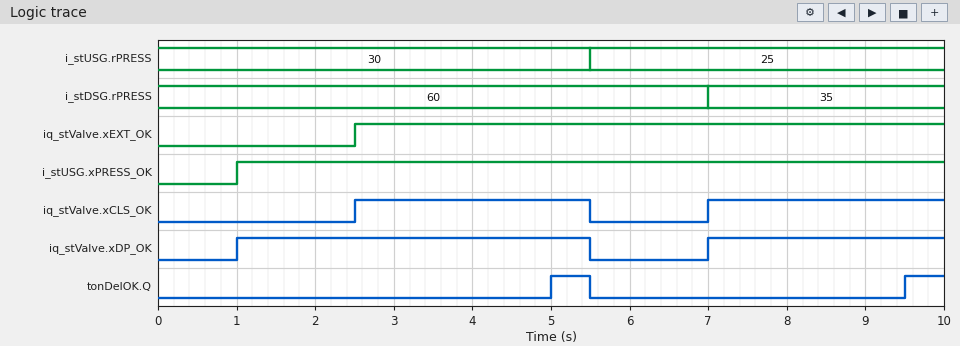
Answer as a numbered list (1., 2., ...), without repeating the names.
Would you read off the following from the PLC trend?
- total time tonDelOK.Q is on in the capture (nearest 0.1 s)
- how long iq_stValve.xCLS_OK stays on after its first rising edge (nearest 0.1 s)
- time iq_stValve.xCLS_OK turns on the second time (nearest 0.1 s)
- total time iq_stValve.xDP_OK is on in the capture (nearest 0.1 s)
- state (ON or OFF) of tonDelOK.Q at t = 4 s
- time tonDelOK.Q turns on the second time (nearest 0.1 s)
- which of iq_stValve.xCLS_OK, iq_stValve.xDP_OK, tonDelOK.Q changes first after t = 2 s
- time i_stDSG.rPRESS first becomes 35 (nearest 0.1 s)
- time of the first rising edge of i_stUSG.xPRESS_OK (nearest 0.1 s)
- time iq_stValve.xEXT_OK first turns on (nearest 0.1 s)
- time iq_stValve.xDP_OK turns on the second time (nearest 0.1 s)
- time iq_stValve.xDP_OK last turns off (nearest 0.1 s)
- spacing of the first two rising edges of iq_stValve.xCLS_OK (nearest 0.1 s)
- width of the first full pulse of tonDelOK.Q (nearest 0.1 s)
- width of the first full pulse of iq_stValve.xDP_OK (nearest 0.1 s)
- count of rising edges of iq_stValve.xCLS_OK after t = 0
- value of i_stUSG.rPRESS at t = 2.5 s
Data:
1. 1.0 s
2. 3.0 s
3. 7.0 s
4. 7.5 s
5. OFF
6. 9.5 s
7. iq_stValve.xCLS_OK
8. 7.0 s
9. 1.0 s
10. 2.5 s
11. 7.0 s
12. 5.5 s
13. 4.5 s
14. 0.5 s
15. 4.5 s
16. 2
17. 30
